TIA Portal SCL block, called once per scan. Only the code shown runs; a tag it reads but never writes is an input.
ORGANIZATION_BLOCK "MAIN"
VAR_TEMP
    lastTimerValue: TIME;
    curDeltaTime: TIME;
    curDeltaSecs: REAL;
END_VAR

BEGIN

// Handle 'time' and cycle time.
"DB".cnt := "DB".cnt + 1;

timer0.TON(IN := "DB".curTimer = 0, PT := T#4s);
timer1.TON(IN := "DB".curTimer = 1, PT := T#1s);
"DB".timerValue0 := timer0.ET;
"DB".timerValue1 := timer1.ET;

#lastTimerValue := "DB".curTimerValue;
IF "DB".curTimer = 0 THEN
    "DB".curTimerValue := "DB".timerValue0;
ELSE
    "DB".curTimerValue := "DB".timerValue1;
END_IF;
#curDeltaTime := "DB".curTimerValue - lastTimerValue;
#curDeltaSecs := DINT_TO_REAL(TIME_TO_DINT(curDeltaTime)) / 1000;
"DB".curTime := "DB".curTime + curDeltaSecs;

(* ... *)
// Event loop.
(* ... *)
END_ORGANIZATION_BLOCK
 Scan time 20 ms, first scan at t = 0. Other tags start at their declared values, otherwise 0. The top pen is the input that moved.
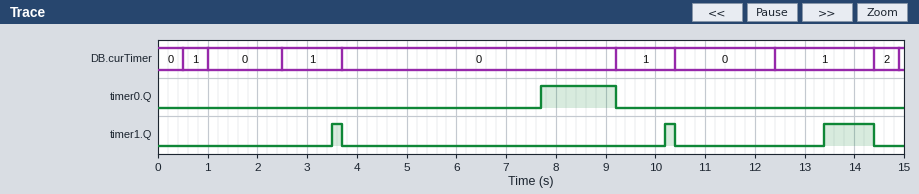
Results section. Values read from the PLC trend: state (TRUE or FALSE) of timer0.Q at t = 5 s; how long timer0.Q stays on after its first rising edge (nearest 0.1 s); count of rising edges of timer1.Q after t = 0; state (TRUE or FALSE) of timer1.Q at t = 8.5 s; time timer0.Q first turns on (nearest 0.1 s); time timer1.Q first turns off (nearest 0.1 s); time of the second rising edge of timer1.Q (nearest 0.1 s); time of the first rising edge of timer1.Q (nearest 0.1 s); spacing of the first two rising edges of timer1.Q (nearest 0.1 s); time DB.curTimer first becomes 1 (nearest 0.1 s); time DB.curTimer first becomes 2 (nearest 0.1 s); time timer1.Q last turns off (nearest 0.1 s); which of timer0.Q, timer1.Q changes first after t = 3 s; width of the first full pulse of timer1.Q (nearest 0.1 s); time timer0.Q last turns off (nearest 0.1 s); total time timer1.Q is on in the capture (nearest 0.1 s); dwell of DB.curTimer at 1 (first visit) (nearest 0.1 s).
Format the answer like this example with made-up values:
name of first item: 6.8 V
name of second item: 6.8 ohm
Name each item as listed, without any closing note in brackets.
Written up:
state (TRUE or FALSE) of timer0.Q at t = 5 s: FALSE
how long timer0.Q stays on after its first rising edge: 1.5 s
count of rising edges of timer1.Q after t = 0: 3
state (TRUE or FALSE) of timer1.Q at t = 8.5 s: FALSE
time timer0.Q first turns on: 7.7 s
time timer1.Q first turns off: 3.7 s
time of the second rising edge of timer1.Q: 10.2 s
time of the first rising edge of timer1.Q: 3.5 s
spacing of the first two rising edges of timer1.Q: 6.7 s
time DB.curTimer first becomes 1: 0.5 s
time DB.curTimer first becomes 2: 14.4 s
time timer1.Q last turns off: 14.4 s
which of timer0.Q, timer1.Q changes first after t = 3 s: timer1.Q
width of the first full pulse of timer1.Q: 0.2 s
time timer0.Q last turns off: 9.2 s
total time timer1.Q is on in the capture: 1.4 s
dwell of DB.curTimer at 1 (first visit): 0.5 s
